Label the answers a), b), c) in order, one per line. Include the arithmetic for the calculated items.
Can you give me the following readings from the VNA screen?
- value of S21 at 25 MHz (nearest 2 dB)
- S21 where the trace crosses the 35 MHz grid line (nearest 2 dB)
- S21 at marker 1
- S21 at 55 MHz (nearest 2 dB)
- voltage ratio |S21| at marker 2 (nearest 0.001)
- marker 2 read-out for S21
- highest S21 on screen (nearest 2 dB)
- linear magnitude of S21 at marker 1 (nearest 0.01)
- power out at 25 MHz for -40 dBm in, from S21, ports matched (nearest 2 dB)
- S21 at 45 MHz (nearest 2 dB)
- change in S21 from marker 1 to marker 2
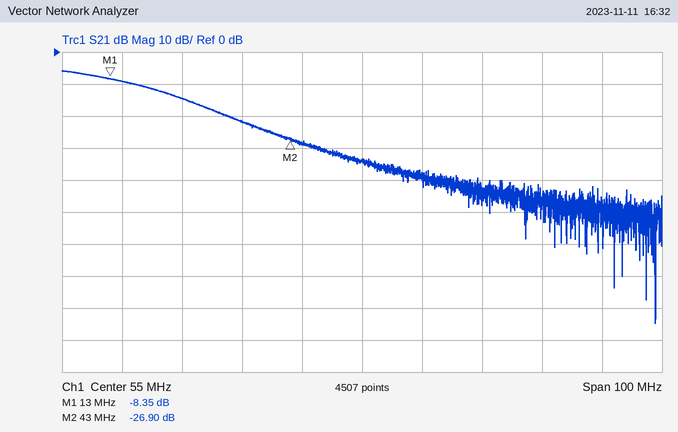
a) -14 dB
b) -22 dB
c) -8.35 dB
d) -34 dB
e) 10^(-26.9/20) ≈ 0.045
f) -26.90 dB
g) -6 dB
h) 10^(-8.35/20) ≈ 0.38
i) -40 dBm + (-14 dB) = -54 dBm
j) -28 dB
k) -26.9 − (-8.35) = -18.55 dB
